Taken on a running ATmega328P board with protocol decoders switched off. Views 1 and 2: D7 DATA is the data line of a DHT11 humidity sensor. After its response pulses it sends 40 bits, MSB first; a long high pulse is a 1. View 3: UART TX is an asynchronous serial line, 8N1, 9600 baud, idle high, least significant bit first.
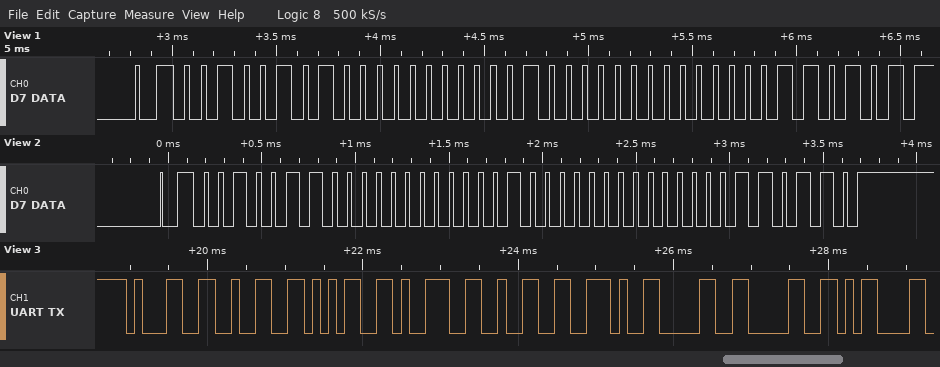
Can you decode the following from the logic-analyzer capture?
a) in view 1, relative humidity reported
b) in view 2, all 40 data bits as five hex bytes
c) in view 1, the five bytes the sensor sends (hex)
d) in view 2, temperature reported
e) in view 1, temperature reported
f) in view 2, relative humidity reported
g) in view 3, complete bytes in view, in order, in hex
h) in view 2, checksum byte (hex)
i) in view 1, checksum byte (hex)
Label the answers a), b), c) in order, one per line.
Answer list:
a) 37 %
b) 26 00 10 00 36
c) 25 00 10 00 35
d) 16.0 °C
e) 16.0 °C
f) 38 %
g) 31 32 35 39 32 2E 30 30 0D
h) 0x36
i) 0x35
